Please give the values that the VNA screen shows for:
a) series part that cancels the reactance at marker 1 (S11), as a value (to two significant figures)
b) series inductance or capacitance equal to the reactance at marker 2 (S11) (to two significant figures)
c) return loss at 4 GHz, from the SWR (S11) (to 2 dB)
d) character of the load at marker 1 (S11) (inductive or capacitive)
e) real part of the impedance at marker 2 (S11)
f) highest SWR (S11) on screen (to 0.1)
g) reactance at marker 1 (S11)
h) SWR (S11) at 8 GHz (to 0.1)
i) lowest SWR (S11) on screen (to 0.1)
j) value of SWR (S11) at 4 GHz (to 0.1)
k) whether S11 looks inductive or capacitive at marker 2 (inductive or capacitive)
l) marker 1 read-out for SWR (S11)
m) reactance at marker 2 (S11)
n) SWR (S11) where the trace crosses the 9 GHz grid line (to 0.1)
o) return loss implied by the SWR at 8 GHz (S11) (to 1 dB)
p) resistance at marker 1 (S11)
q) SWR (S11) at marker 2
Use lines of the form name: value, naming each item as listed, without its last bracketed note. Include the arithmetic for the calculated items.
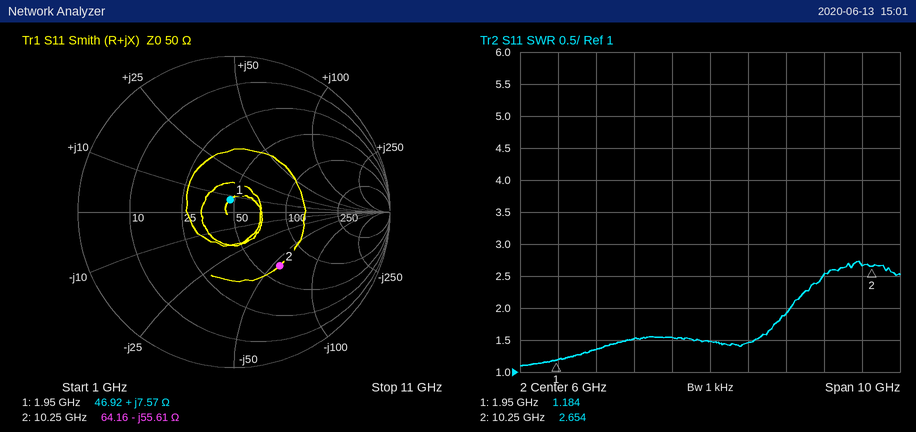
series part that cancels the reactance at marker 1 (S11), as a value: C = 1/(2π × 1.95 GHz × 7.57 Ω) ≈ 11 pF
series inductance or capacitance equal to the reactance at marker 2 (S11): C = 1/(2π × 10.25 GHz × 55.61 Ω) ≈ 279 fF, so 280 fF to two significant figures
return loss at 4 GHz, from the SWR (S11): −20 log10((1.5 − 1)/(1.5 + 1)) ≈ 14 dB
character of the load at marker 1 (S11): inductive
real part of the impedance at marker 2: 64.16 Ω
highest SWR (S11) on screen: 2.7
reactance at marker 1: +7.57 Ω
SWR (S11) at 8 GHz: 1.9
lowest SWR (S11) on screen: 1.1
value of SWR (S11) at 4 GHz: 1.5
whether S11 looks inductive or capacitive at marker 2: capacitive
marker 1 read-out for SWR: 1.184
reactance at marker 2: -55.61 Ω
SWR (S11) where the trace crosses the 9 GHz grid line: 2.5
return loss implied by the SWR at 8 GHz (S11): −20 log10((1.9 − 1)/(1.9 + 1)) ≈ 10 dB
resistance at marker 1: 46.92 Ω
SWR (S11) at marker 2: 2.654
